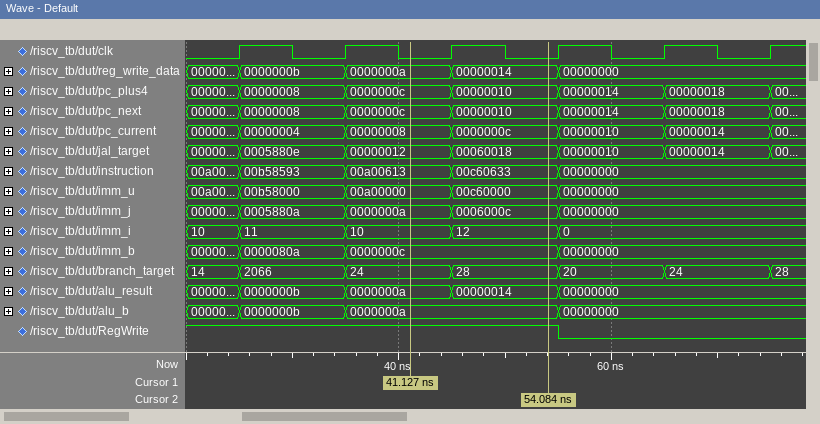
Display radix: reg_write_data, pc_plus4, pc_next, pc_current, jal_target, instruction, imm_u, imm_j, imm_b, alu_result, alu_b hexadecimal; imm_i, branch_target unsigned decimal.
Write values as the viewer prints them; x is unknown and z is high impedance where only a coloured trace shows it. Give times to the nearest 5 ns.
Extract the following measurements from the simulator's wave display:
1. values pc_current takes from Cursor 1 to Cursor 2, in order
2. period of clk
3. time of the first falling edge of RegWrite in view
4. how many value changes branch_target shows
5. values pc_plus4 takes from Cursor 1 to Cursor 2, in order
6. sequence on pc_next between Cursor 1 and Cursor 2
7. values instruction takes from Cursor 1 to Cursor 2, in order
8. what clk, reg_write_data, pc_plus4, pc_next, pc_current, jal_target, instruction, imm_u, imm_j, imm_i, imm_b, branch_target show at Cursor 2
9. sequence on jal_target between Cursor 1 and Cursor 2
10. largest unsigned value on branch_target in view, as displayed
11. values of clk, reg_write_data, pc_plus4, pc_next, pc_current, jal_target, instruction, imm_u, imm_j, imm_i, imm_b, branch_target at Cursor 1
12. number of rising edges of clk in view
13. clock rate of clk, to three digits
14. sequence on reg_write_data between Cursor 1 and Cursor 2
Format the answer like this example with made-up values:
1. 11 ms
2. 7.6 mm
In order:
1. 00000008, 0000000c
2. 10 ns
3. 55 ns
4. 6
5. 0000000c, 00000010
6. 0000000c, 00000010
7. 00a00613, 00c60633
8. clk=0, reg_write_data=00000014, pc_plus4=00000010, pc_next=00000010, pc_current=0000000c, jal_target=00060018, instruction=00c60633, imm_u=00c60000, imm_j=0006000c, imm_i=12, imm_b=0000000c, branch_target=28
9. 00000012, 00060018
10. 2066
11. clk=0, reg_write_data=0000000a, pc_plus4=0000000c, pc_next=0000000c, pc_current=00000008, jal_target=00000012, instruction=00a00613, imm_u=00a00000, imm_j=0000000a, imm_i=10, imm_b=0000000c, branch_target=24
12. 6
13. 100 MHz
14. 0000000a, 00000014
